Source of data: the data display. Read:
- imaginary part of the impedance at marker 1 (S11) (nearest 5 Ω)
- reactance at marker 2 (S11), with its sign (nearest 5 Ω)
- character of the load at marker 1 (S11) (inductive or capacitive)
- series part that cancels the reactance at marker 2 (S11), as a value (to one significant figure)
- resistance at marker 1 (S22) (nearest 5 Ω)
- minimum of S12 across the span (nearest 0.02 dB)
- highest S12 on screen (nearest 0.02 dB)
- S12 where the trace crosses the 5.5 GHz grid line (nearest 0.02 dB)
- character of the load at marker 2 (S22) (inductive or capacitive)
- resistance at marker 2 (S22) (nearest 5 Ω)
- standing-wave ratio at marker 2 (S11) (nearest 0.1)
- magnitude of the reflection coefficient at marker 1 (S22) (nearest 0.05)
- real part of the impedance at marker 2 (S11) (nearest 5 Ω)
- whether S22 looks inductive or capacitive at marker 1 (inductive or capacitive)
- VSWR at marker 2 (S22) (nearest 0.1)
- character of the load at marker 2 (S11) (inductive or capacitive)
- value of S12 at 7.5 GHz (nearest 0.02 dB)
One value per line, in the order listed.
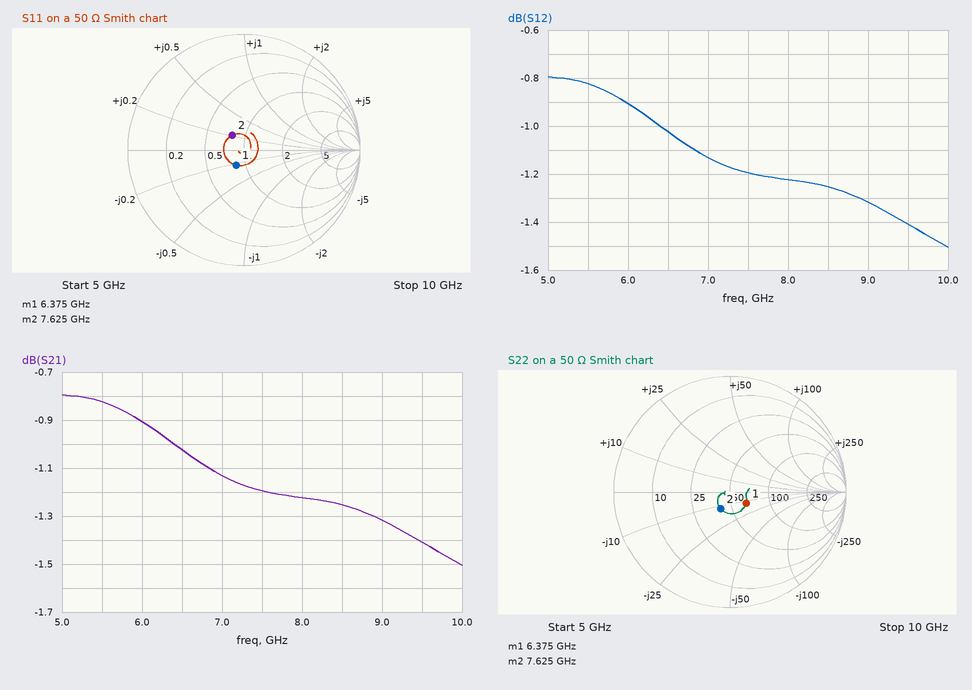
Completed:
-10 Ω
+10 Ω
capacitive
2 pF
65 Ω
-1.50 dB
-0.80 dB
-0.82 dB
capacitive
40 Ω
1.4
0.15
40 Ω
capacitive
1.4
inductive
-1.20 dB
